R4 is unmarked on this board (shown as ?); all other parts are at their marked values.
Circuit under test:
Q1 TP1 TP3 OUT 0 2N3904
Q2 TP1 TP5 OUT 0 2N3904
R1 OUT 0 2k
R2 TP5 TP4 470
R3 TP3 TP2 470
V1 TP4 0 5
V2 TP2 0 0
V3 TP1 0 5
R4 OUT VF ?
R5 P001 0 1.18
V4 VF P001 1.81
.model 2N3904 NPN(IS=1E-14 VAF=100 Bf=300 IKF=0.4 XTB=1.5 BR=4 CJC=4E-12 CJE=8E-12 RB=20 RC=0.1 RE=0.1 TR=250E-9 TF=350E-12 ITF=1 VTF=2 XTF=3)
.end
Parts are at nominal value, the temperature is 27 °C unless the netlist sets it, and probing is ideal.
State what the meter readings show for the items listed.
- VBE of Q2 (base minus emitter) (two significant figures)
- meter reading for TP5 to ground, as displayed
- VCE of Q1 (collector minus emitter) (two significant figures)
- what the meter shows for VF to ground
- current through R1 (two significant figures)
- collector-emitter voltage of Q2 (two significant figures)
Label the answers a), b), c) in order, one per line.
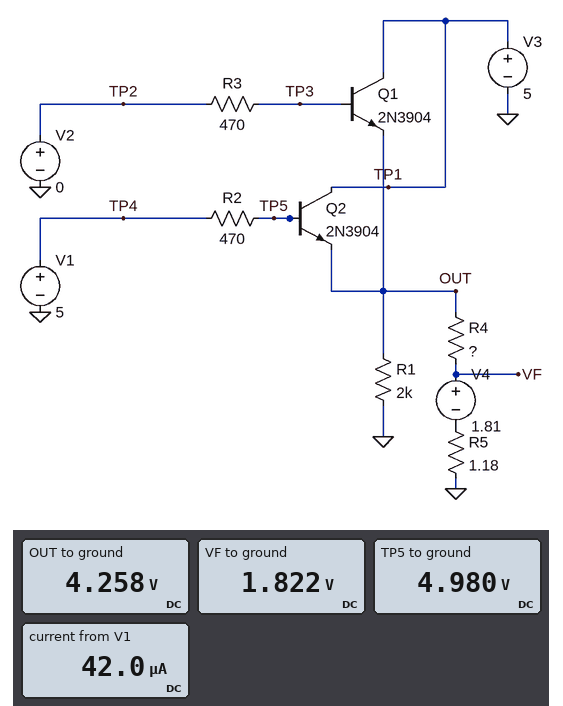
a) 720 mV
b) 4.980 V
c) 740 mV
d) 1.822 V
e) 2.1 mA
f) 740 mV
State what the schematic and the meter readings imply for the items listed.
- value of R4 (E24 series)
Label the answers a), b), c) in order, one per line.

a) 240 Ω
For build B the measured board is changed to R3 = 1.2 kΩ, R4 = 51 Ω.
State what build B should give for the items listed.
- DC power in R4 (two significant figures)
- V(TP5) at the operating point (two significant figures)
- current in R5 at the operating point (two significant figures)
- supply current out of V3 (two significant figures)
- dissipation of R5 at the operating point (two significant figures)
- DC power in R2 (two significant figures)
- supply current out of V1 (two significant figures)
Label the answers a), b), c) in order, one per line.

a) 100 mW
b) 4.9 V
c) 45 mA
d) 47 mA
e) 2.4 mW
f) 14 µW
g) 170 µA
